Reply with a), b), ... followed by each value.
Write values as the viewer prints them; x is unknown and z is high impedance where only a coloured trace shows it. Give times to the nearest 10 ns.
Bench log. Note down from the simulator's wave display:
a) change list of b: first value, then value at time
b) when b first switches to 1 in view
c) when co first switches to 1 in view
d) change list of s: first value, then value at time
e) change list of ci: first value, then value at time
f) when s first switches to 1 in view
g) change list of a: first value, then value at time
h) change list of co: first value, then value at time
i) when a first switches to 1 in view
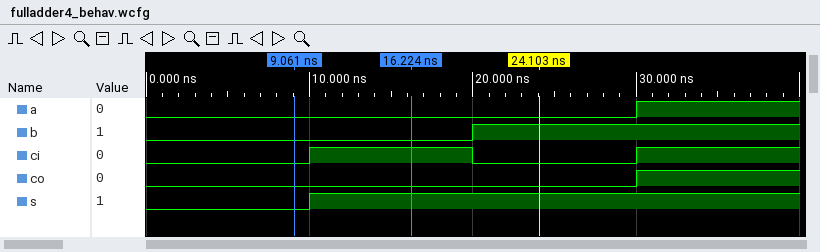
a) 0, 1 at 20 ns
b) 20 ns
c) 30 ns
d) 0, 1 at 10 ns
e) 0, 1 at 10 ns, 0 at 20 ns, 1 at 30 ns
f) 10 ns
g) 0, 1 at 30 ns
h) 0, 1 at 30 ns
i) 30 ns
